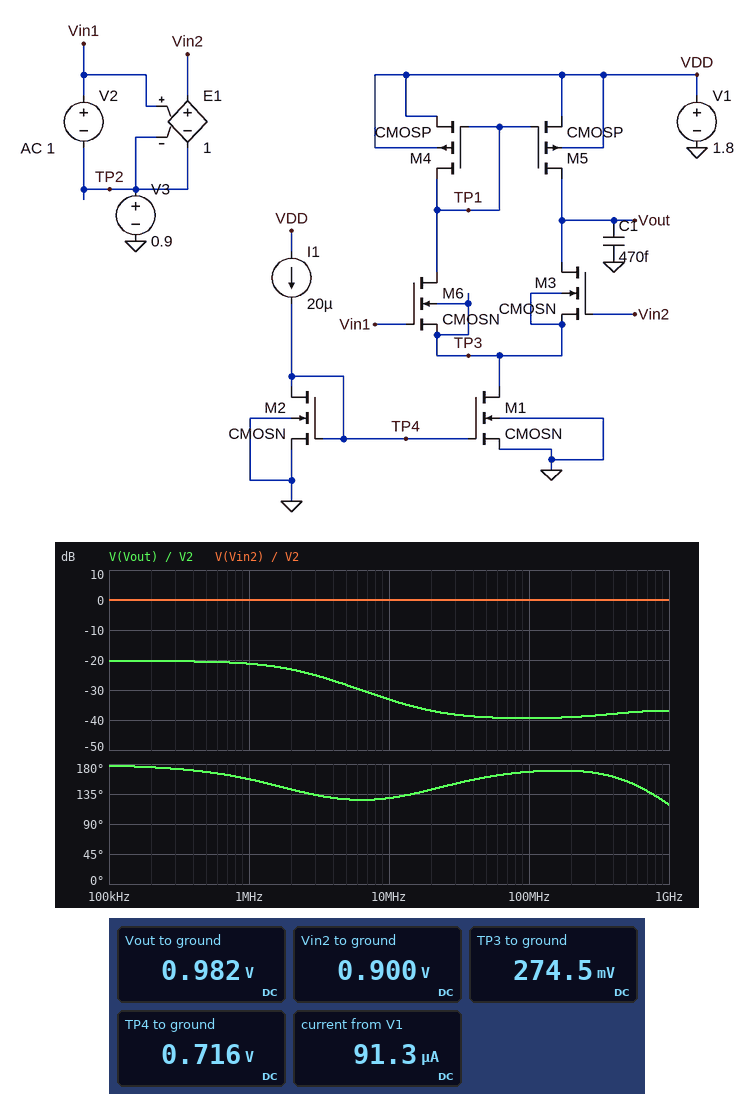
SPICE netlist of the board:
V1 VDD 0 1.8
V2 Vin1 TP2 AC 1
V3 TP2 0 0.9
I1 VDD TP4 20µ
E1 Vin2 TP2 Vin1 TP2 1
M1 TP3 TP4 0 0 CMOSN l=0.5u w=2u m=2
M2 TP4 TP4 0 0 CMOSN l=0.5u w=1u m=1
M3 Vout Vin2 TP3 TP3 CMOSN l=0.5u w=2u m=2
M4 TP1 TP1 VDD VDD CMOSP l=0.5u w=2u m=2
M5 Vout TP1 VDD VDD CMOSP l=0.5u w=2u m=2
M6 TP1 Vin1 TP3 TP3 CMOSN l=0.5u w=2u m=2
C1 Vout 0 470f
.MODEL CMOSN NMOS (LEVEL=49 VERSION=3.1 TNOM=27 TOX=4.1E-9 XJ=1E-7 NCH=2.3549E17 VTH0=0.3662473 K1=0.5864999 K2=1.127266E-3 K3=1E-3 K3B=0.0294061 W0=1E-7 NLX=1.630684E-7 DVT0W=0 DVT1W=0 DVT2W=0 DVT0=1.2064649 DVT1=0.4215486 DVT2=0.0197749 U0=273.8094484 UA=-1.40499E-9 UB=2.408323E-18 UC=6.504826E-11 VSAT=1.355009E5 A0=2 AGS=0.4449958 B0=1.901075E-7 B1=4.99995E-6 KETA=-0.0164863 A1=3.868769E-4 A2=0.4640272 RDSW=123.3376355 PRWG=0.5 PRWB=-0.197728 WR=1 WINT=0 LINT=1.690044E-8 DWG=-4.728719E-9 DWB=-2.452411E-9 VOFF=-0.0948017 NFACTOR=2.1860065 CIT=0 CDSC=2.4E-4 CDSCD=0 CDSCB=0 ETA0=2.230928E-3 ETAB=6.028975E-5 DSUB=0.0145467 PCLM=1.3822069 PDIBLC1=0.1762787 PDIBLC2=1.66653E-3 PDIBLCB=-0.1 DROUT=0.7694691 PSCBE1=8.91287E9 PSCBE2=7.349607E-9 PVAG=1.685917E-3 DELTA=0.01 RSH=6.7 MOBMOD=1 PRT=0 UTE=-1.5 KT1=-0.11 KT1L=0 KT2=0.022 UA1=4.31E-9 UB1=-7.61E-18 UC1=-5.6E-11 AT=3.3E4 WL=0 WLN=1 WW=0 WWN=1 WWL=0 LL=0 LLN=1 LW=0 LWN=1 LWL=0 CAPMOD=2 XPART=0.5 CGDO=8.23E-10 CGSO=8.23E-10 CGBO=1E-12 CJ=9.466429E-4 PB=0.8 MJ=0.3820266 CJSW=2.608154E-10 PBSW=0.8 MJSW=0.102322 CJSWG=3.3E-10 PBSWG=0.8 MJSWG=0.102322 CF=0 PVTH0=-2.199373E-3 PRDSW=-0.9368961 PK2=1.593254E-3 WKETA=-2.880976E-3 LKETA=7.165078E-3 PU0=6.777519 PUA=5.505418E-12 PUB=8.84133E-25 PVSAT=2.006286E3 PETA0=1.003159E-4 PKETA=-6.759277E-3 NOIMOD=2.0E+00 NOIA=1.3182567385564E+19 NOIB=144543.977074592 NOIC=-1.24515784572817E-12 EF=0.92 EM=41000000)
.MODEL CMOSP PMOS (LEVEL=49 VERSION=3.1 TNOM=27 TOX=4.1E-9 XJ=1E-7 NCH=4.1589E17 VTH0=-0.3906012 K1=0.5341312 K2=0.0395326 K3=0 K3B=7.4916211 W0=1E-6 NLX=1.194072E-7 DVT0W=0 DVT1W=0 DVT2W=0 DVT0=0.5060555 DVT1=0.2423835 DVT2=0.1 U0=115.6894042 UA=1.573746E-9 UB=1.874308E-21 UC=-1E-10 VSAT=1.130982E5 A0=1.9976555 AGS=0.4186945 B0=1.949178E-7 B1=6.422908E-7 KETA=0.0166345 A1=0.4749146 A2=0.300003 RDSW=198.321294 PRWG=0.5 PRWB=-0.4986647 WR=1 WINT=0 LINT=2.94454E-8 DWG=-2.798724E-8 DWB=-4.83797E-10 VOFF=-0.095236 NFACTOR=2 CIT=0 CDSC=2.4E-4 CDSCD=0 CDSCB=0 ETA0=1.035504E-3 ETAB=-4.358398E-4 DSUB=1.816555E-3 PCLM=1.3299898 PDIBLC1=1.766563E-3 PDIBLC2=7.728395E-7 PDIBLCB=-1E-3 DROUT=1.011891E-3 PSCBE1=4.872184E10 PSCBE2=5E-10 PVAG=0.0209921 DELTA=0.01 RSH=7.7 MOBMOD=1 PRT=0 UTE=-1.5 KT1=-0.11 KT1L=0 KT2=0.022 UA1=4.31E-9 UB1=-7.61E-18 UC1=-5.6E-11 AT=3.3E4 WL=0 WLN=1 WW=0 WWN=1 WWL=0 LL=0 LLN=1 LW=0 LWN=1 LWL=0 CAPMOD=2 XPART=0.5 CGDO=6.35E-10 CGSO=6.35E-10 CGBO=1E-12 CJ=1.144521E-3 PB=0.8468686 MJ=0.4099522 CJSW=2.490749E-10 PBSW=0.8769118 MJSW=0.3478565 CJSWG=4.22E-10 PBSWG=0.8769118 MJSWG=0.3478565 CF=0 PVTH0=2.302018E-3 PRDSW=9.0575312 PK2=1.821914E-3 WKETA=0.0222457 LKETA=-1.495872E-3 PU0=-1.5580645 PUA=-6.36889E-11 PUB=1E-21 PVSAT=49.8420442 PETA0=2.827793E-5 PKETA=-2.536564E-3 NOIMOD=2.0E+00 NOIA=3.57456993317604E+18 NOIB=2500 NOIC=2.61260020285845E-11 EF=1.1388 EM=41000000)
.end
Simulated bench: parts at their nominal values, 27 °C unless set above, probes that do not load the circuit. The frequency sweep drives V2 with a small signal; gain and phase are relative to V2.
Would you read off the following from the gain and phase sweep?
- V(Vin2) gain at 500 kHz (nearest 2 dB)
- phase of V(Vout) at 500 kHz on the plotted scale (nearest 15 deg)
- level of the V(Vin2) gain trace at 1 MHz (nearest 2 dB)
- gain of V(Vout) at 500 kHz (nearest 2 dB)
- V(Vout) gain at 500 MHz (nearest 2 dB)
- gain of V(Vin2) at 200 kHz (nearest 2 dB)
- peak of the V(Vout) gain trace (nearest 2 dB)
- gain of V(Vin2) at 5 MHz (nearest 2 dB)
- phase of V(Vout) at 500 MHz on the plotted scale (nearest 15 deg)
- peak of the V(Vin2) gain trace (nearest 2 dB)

0 dB
165 deg
0 dB
-20 dB
-38 dB
0 dB
-20 dB
0 dB
150 deg
0 dB
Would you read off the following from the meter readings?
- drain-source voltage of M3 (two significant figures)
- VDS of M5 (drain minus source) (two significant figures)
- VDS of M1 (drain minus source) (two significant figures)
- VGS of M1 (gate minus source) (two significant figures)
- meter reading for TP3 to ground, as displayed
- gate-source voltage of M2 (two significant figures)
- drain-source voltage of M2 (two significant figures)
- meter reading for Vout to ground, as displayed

710 mV
-820 mV
270 mV
720 mV
274.5 mV
720 mV
720 mV
0.982 V
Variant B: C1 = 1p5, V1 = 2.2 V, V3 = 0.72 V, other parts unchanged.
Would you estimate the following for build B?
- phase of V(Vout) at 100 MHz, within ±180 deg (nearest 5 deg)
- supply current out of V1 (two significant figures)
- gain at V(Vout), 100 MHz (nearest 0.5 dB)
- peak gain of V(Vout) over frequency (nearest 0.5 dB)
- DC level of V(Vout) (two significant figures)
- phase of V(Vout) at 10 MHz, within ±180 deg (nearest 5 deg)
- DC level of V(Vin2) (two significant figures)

160 deg
74 µA
-36.0 dB
-4.5 dB
1.4 V
120 deg
720 mV
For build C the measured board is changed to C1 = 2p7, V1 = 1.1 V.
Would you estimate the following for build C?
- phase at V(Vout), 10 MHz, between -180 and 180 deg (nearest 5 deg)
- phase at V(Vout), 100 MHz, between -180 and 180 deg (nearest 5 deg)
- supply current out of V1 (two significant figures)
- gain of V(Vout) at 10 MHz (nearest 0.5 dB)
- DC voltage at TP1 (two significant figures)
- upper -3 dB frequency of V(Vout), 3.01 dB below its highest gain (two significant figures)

135 deg
65 deg
88 µA
-26.0 dB
290 mV
11 MHz
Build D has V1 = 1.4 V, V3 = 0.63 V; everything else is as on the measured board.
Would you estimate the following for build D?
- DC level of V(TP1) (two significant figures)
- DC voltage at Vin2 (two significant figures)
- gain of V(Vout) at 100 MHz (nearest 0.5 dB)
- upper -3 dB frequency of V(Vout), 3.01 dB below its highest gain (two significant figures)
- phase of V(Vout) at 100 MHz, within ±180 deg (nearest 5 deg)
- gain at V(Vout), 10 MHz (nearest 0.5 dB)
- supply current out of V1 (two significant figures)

710 mV
630 mV
-22.5 dB
1.3 MHz
160 deg
-17.5 dB
54 µA
